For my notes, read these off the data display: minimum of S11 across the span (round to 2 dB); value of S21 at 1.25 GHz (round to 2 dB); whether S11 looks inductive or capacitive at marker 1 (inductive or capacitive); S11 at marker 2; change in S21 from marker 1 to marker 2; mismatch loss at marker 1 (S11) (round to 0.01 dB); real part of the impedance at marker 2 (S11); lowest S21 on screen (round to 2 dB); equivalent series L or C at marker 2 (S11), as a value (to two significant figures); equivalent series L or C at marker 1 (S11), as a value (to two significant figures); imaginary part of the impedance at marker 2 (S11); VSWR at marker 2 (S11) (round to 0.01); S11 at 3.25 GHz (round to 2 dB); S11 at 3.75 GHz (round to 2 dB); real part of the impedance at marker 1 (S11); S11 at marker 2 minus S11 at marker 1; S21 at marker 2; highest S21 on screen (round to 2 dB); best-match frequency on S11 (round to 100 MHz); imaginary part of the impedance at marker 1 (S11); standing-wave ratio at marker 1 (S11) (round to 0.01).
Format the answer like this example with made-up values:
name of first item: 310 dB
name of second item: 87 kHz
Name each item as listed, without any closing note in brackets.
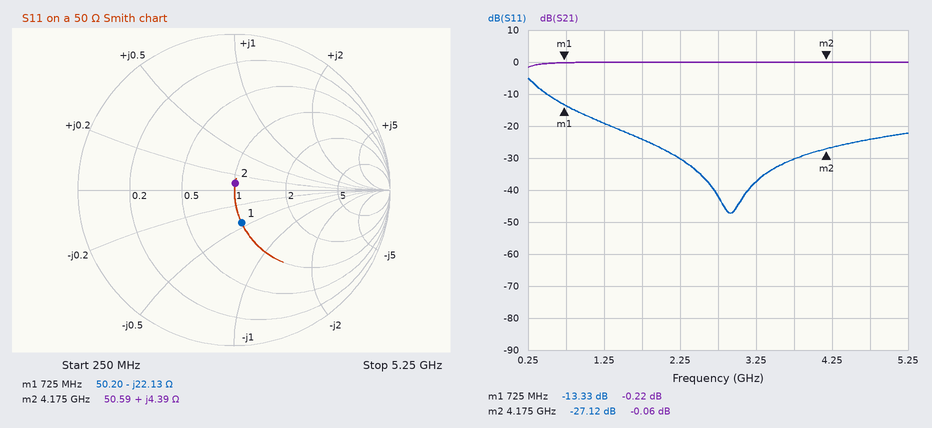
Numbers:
minimum of S11 across the span: -48 dB
value of S21 at 1.25 GHz: 0 dB
whether S11 looks inductive or capacitive at marker 1: capacitive
S11 at marker 2: -27.12 dB
change in S21 from marker 1 to marker 2: 0.16 dB
mismatch loss at marker 1 (S11): 0.21 dB
real part of the impedance at marker 2: 50.59 Ω
lowest S21 on screen: -2 dB
equivalent series L or C at marker 2 (S11), as a value: 170 pH
equivalent series L or C at marker 1 (S11), as a value: 9.9 pF
imaginary part of the impedance at marker 2: +4.39 Ω
VSWR at marker 2 (S11): 1.09
S11 at 3.25 GHz: -38 dB
S11 at 3.75 GHz: -30 dB
real part of the impedance at marker 1: 50.20 Ω
S11 at marker 2 minus S11 at marker 1: -13.79 dB
S21 at marker 2: -0.06 dB
highest S21 on screen: 0 dB
best-match frequency on S11: 2.9 GHz
imaginary part of the impedance at marker 1: -22.13 Ω
standing-wave ratio at marker 1 (S11): 1.55
